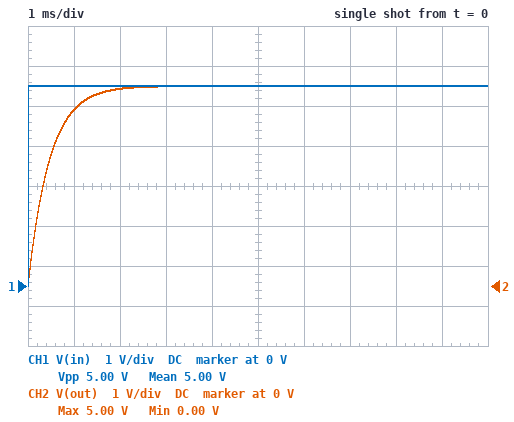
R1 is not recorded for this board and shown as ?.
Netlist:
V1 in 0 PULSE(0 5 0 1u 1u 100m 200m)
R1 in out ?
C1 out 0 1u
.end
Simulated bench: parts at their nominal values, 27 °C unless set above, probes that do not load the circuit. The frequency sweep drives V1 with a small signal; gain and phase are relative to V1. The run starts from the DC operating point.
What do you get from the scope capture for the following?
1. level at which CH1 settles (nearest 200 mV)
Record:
5.0 V
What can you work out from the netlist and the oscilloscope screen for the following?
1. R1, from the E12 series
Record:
470 Ω
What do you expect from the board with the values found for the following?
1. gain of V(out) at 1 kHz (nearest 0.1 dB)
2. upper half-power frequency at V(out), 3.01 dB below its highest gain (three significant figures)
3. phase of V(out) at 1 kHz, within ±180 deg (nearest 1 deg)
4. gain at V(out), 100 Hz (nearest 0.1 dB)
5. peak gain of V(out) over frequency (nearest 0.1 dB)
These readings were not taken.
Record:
-9.9 dB
339 Hz
-71 deg
-0.4 dB
0 dB
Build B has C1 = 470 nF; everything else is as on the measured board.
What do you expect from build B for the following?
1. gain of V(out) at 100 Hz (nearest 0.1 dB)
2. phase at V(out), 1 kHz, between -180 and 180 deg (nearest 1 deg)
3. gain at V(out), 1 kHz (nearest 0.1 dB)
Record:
-0.1 dB
-54 deg
-4.7 dB
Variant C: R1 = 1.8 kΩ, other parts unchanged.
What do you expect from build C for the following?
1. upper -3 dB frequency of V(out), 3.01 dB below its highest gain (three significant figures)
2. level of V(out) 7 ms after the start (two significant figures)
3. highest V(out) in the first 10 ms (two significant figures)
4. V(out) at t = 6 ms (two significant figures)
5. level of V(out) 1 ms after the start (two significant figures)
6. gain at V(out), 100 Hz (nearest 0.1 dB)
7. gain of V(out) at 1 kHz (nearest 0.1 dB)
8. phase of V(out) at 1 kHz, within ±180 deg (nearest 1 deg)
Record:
88.4 Hz
4.9 V
5.0 V
4.8 V
2.1 V
-3.6 dB
-21.1 dB
-85 deg
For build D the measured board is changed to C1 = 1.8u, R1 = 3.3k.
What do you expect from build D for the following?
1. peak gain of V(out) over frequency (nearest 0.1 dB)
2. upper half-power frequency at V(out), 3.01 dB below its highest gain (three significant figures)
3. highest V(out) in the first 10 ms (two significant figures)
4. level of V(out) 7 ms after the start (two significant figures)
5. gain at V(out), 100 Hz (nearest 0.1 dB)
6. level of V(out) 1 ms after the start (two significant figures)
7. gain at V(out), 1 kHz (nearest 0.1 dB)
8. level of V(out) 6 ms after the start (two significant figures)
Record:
0 dB
26.8 Hz
4.1 V
3.5 V
-11.7 dB
770 mV
-31.4 dB
3.2 V
